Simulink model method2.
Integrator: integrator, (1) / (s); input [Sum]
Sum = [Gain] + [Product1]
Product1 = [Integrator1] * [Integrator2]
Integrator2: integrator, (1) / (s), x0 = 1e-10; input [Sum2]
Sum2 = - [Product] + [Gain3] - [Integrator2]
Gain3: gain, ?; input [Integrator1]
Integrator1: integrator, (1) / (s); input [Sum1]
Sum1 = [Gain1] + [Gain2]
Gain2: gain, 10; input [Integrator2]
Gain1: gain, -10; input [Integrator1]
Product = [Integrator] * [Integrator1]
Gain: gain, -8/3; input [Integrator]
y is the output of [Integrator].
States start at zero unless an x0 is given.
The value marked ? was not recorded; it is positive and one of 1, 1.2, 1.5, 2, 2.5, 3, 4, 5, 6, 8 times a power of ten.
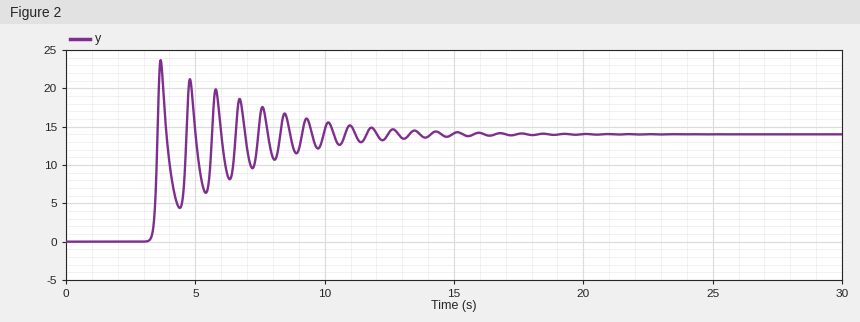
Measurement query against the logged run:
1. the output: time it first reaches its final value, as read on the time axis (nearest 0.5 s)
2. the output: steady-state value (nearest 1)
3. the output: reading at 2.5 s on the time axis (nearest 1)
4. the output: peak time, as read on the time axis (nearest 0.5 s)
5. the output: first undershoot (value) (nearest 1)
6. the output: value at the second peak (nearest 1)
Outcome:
3.5 s
14
0
3.5 s
4
21
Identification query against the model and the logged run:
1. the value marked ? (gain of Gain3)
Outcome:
15
